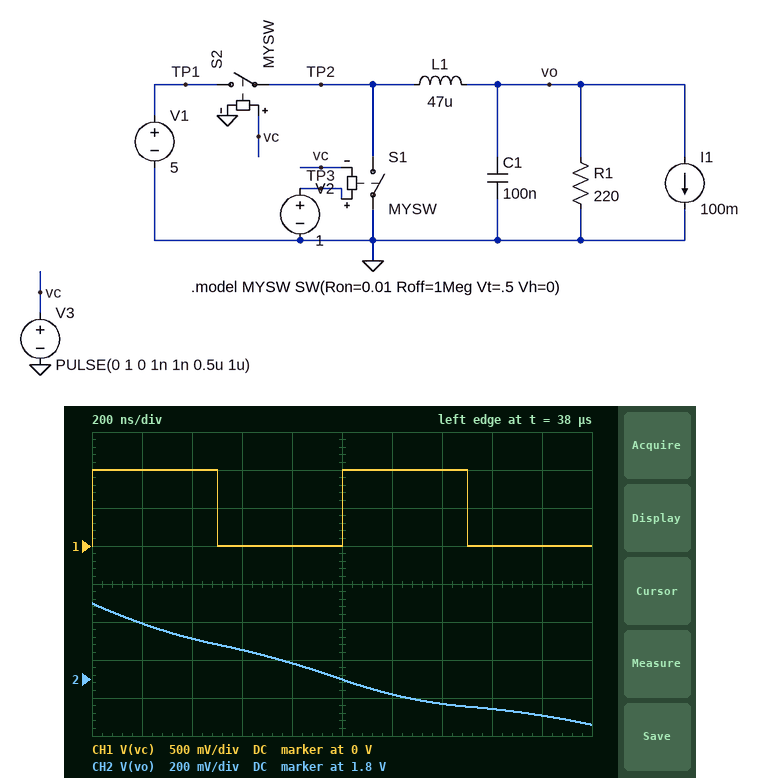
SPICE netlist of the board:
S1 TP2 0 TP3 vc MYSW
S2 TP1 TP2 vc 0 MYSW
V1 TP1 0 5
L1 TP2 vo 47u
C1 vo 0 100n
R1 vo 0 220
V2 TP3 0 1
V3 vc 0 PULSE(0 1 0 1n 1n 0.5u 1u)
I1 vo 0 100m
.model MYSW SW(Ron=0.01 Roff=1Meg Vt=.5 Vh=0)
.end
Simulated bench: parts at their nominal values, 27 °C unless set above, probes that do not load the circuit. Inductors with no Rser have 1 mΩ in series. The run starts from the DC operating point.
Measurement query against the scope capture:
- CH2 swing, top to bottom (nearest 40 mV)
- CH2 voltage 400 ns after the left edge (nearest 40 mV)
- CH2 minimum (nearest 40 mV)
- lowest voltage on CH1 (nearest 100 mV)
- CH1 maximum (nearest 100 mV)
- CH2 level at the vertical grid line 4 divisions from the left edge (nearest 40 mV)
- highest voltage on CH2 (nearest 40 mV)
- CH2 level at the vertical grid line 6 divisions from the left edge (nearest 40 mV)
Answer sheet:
640 mV
2.00 V
1.56 V
0 V
1.0 V
1.88 V
2.20 V
1.72 V
